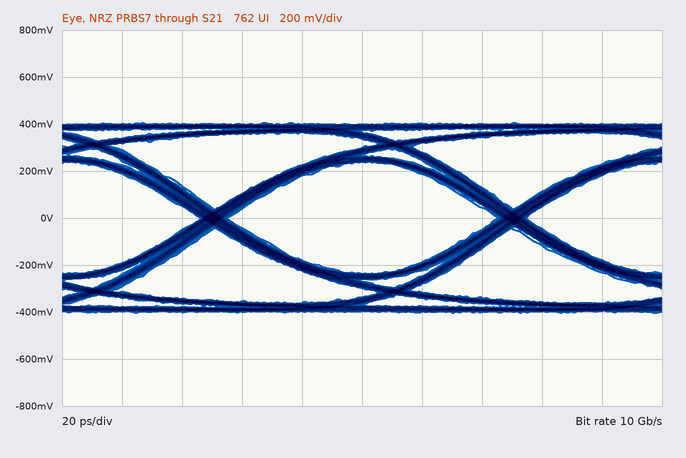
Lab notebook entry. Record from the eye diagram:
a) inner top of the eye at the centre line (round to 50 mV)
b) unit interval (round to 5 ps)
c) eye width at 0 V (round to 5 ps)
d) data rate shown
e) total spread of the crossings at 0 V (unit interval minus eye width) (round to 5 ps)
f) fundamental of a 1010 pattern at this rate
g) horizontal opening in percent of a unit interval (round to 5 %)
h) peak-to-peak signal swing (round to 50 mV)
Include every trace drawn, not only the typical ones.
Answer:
250 mV
100 ps
90 ps
10 Gb/s
10 ps
5 GHz
90 %
800 mV
